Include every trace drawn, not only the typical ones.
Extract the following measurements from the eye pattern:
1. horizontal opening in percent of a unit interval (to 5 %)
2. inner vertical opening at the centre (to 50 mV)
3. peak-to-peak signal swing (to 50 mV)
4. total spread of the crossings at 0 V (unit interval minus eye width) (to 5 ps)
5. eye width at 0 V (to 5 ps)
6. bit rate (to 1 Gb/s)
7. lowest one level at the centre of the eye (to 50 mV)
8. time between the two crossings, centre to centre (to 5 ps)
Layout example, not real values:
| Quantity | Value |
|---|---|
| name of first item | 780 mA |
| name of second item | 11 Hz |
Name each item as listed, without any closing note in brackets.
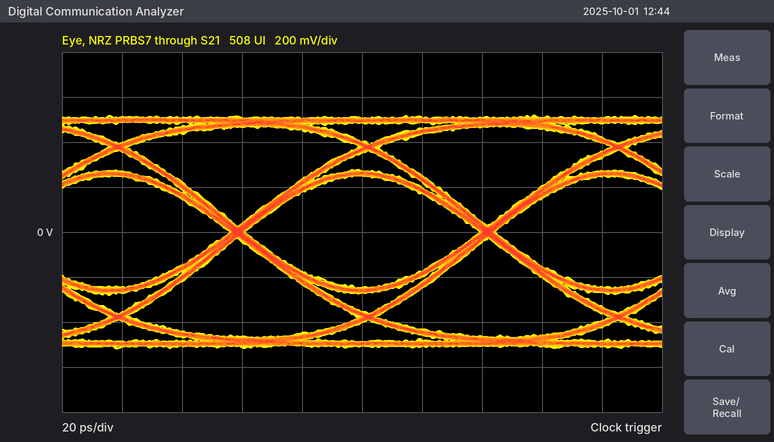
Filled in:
| Quantity | Value |
|---|---|
| horizontal opening in percent of a unit interval | 95 % |
| inner vertical opening at the centre | 500 mV |
| peak-to-peak signal swing | 1.05 V |
| total spread of the crossings at 0 V (unit interval minus eye width) | 5 ps |
| eye width at 0 V | 80 ps |
| bit rate | 12 Gb/s |
| lowest one level at the centre of the eye | 250 mV |
| time between the two crossings, centre to centre | 85 ps |
